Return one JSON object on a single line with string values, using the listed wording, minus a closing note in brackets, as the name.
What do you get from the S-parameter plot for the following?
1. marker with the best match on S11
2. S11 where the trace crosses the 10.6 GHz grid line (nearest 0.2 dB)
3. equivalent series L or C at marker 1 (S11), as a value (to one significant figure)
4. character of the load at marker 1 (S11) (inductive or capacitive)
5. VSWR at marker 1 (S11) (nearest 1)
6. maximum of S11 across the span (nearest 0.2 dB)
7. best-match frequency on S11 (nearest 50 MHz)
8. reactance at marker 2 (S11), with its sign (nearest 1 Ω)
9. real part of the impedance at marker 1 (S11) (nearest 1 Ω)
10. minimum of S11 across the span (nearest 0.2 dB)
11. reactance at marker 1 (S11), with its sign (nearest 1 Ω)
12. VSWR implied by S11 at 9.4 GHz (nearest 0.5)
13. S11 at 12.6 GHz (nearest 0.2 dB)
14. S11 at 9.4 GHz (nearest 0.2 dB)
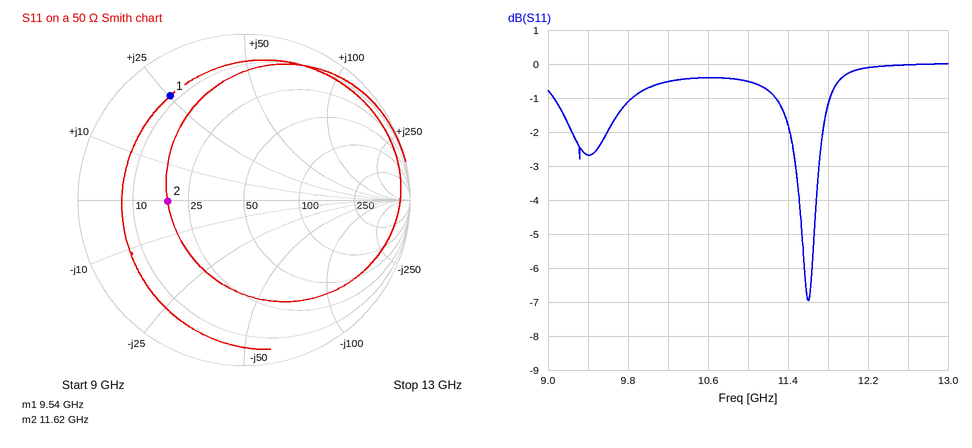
{"marker with the best match on S11": "marker 2", "S11 where the trace crosses the 10.6 GHz grid line": "-0.4 dB", "equivalent series L or C at marker 1 (S11), as a value": "400 pH", "character of the load at marker 1 (S11)": "inductive", "VSWR at marker 1 (S11)": "8", "maximum of S11 across the span": "0.0 dB", "best-match frequency on S11": "11.60 GHz", "reactance at marker 2 (S11), with its sign": "0 Ω", "real part of the impedance at marker 1 (S11)": "8 Ω", "minimum of S11 across the span": "-7.0 dB", "reactance at marker 1 (S11), with its sign": "+25 Ω", "VSWR implied by S11 at 9.4 GHz": "6.5", "S11 at 12.6 GHz": "0.0 dB", "S11 at 9.4 GHz": "-2.6 dB"}
